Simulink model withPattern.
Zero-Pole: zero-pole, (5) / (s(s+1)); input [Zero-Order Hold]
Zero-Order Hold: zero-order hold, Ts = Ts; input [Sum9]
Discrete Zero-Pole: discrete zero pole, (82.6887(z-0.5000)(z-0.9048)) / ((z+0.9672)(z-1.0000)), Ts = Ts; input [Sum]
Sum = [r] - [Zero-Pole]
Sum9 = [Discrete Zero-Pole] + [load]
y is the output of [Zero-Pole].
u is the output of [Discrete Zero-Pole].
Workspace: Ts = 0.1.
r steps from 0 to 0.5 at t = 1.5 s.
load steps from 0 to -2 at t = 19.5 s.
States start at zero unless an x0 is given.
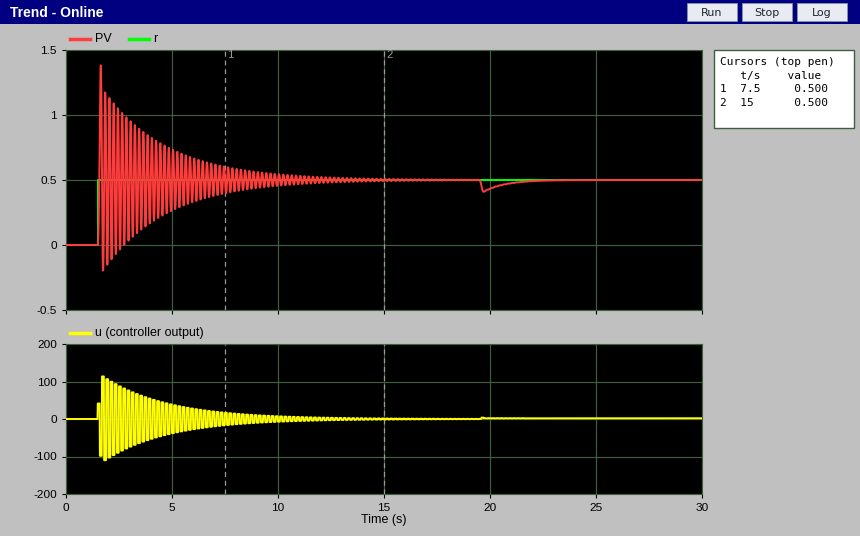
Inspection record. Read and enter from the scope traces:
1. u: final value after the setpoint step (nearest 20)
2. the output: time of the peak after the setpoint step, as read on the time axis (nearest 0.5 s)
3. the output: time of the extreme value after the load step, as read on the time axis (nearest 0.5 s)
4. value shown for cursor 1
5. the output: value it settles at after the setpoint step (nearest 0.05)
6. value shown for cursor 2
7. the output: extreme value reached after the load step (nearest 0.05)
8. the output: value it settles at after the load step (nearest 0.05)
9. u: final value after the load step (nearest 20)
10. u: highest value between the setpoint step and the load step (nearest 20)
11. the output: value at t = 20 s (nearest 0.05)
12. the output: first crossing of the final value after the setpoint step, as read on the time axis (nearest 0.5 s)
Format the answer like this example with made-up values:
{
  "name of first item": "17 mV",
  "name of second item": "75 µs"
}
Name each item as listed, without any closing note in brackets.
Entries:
{
  "u: final value after the setpoint step": "0",
  "the output: time of the peak after the setpoint step, as read on the time axis": "1.5 s",
  "the output: time of the extreme value after the load step, as read on the time axis": "19.5 s",
  "value shown for cursor 1": "0.500",
  "the output: value it settles at after the setpoint step": "0.50",
  "value shown for cursor 2": "0.500",
  "the output: extreme value reached after the load step": "0.40",
  "the output: value it settles at after the load step": "0.50",
  "u: final value after the load step": "0",
  "u: highest value between the setpoint step and the load step": "120",
  "the output: value at t = 20 s": "0.45",
  "the output: first crossing of the final value after the setpoint step, as read on the time axis": "1.5 s"
}
